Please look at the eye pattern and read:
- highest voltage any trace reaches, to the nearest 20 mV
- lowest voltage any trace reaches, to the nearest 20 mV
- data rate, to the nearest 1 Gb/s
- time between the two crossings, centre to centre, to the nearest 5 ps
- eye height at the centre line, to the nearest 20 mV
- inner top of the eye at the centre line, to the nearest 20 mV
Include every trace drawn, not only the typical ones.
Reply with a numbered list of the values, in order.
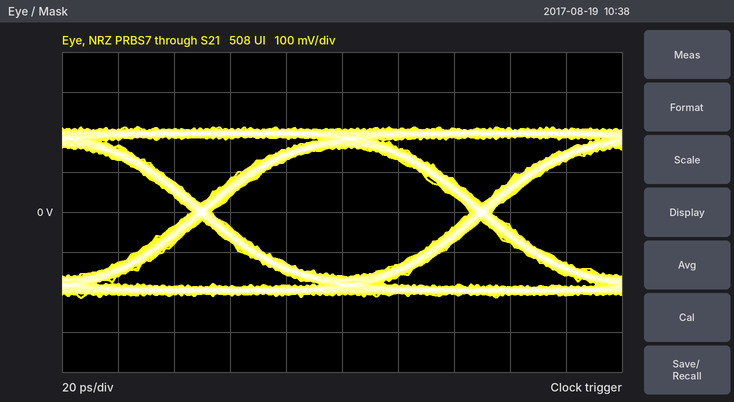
1. 220 mV
2. -220 mV
3. 10 Gb/s
4. 100 ps
5. 320 mV
6. 160 mV
